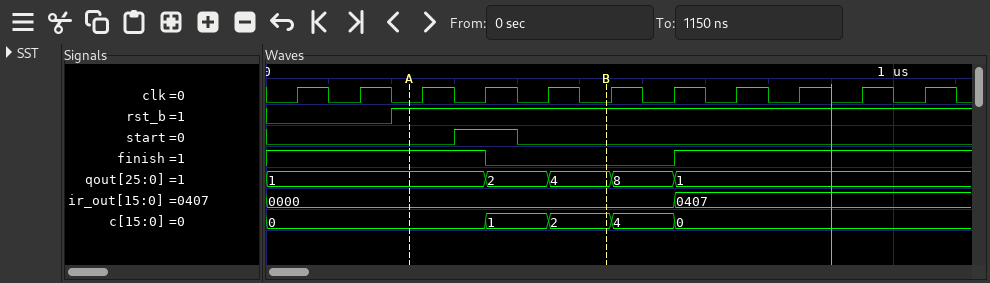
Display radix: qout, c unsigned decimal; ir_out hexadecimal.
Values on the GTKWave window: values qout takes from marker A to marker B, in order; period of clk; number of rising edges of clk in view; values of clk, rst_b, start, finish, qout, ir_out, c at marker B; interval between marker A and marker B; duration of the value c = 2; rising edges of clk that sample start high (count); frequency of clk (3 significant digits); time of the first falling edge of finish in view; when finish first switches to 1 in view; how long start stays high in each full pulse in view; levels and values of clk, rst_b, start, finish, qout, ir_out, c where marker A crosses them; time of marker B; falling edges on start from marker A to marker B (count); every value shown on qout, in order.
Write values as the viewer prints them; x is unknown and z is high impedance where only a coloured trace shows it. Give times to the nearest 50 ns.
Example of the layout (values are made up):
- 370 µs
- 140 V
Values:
- 1, 2, 4
- 100 ns
- 11
- clk=0, rst_b=1, start=0, finish=0, qout=4, ir_out=0000, c=2
- 300 ns
- 100 ns
- 1
- 10.0 MHz
- 350 ns
- 650 ns
- 100 ns
- clk=0, rst_b=1, start=0, finish=1, qout=1, ir_out=0000, c=0
- 550 ns
- 1
- 1, 2, 4, 8, 1
